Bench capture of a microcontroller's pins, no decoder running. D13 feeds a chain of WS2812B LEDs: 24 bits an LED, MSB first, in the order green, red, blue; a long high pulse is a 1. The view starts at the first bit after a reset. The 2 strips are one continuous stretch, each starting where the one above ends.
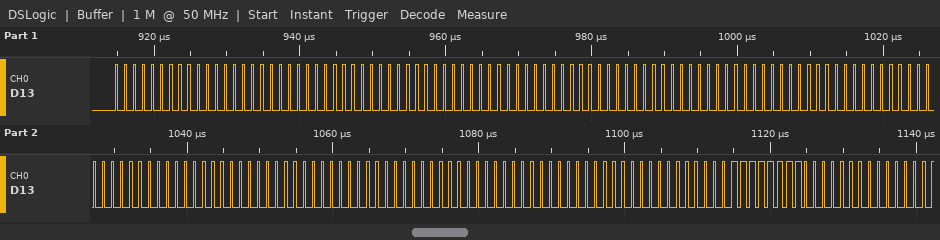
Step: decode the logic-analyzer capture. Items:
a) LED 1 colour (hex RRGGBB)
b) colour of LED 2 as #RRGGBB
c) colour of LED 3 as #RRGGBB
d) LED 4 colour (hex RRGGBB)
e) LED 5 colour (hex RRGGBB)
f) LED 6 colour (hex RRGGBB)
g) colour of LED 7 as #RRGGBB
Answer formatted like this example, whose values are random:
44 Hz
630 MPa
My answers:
#000000
#000000
#000000
#000000
#000000
#000000
#0000FF
